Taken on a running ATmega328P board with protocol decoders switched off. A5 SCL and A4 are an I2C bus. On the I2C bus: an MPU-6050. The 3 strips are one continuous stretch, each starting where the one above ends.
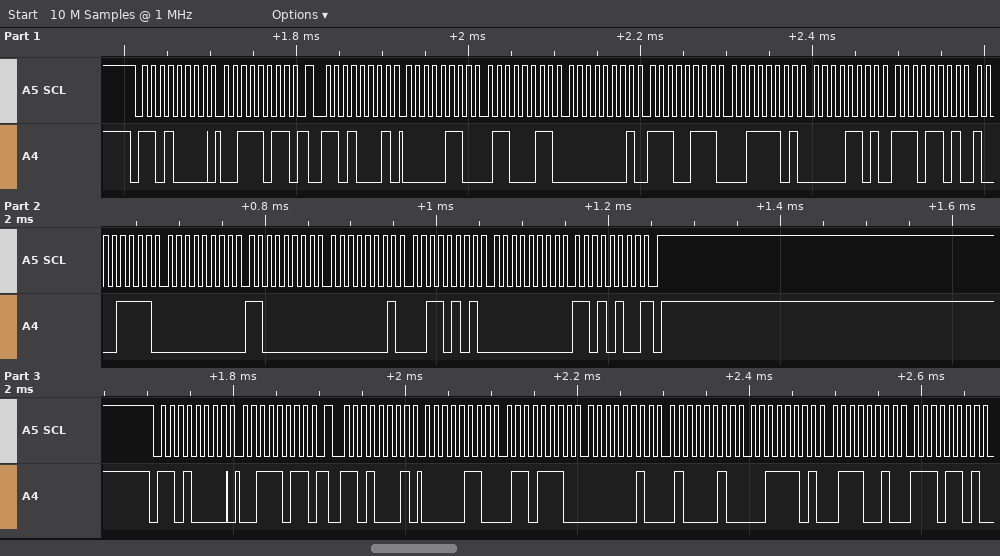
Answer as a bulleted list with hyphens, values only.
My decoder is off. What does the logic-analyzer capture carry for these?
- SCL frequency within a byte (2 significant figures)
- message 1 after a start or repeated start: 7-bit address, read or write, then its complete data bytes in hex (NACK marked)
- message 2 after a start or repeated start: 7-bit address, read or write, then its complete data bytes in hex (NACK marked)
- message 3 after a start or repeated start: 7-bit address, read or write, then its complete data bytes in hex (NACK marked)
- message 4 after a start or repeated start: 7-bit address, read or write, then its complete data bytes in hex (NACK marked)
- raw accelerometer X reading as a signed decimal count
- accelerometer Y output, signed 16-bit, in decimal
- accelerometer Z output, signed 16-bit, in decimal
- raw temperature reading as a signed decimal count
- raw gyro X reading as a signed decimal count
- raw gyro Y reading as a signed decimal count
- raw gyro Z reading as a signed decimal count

- 100 kHz
- 0x68 write: 3B
- 0x68 read: 06 63 01 E7 3D 0D ED 8F 00 C0 01 35 00 D4 NACK
- 0x68 write: 3B
- 0x68 read: 06 6E 02 42 3D 72 ED
- 1635
- 487
- 15629
- -4721
- 192
- 309
- 212
